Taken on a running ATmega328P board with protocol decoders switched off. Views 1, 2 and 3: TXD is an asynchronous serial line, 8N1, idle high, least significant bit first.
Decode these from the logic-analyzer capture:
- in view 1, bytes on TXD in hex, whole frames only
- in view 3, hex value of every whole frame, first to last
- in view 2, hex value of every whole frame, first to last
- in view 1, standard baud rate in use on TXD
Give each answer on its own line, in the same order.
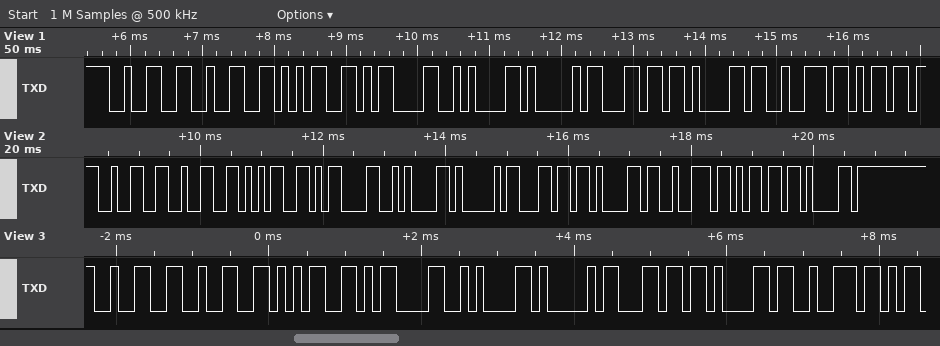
32 32 35 0D 0A 41 6C 61 72 6D
0x32 0x32 0x35 0x0D 0x0A 0x41 0x6C 0x61 0x72
0x32 0x32 0x35 0x0D 0x0A 0x41 0x6C 0x61 0x72 0x6D 0x61
9600 baud
